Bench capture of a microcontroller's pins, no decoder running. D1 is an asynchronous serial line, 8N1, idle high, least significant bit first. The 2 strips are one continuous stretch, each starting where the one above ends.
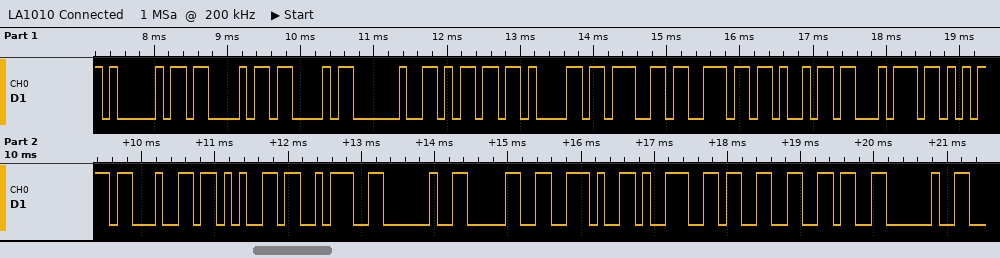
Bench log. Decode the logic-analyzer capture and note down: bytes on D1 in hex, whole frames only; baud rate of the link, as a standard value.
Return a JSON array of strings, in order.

["41 43 43 20 6D 61 67 6E 69 74 75 64 65 3A 20 30 2E 39 33 36 20", "9600 baud"]
